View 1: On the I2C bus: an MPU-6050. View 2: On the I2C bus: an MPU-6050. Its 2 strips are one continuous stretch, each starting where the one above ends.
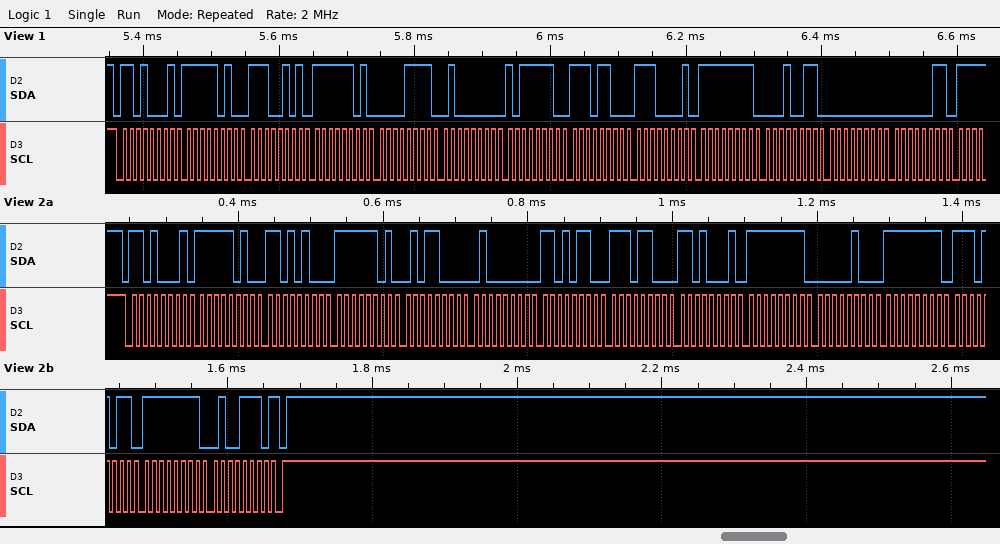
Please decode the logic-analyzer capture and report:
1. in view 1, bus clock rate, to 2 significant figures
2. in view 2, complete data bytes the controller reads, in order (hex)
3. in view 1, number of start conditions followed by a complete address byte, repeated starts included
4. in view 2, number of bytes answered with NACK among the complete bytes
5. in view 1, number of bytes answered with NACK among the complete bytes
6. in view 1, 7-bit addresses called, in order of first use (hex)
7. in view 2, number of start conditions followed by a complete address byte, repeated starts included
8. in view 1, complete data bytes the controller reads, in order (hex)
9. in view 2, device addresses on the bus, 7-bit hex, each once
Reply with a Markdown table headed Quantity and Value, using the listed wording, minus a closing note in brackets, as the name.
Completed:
| Quantity | Value |
|---|---|
| in view 1, bus clock rate, to 2 significant figures | 100 kHz |
| in view 2, complete data bytes the controller reads, in order | FA D4 FD 58 40 D6 EC D1 FF 04 FF EB FF 4E |
| in view 1, number of start conditions followed by a complete address byte, repeated starts included | 1 |
| in view 2, number of bytes answered with NACK among the complete bytes | 1 |
| in view 1, number of bytes answered with NACK among the complete bytes | 0 |
| in view 1, 7-bit addresses called, in order of first use | 0x68 |
| in view 2, number of start conditions followed by a complete address byte, repeated starts included | 1 |
| in view 1, complete data bytes the controller reads, in order | FA E5 FD 0F 40 BE EC E1 FF 13 00 03 |
| in view 2, device addresses on the bus, 7-bit hex, each once | 0x68 |
